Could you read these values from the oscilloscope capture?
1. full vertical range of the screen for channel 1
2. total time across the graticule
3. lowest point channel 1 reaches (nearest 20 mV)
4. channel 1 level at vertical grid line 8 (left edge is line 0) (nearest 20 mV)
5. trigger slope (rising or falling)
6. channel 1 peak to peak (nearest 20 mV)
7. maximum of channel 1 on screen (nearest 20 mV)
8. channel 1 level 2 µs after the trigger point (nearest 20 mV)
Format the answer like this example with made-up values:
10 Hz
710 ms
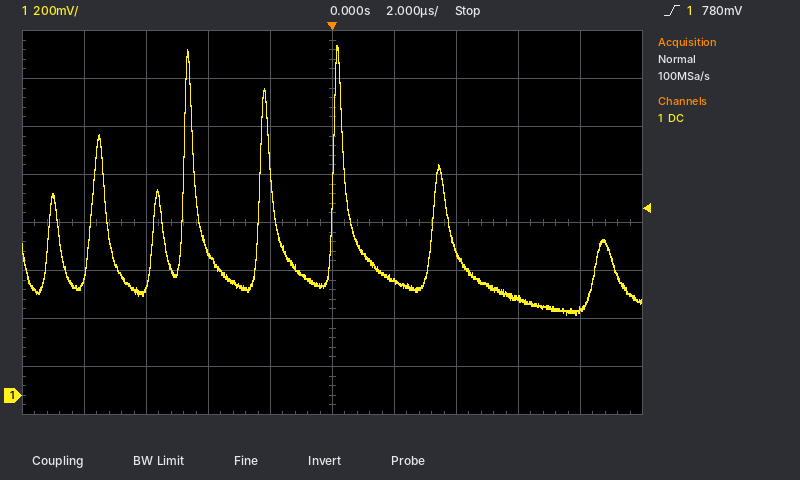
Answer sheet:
1.6 V
20 µs
340 mV
400 mV
rising
1.12 V
1.46 V
480 mV
